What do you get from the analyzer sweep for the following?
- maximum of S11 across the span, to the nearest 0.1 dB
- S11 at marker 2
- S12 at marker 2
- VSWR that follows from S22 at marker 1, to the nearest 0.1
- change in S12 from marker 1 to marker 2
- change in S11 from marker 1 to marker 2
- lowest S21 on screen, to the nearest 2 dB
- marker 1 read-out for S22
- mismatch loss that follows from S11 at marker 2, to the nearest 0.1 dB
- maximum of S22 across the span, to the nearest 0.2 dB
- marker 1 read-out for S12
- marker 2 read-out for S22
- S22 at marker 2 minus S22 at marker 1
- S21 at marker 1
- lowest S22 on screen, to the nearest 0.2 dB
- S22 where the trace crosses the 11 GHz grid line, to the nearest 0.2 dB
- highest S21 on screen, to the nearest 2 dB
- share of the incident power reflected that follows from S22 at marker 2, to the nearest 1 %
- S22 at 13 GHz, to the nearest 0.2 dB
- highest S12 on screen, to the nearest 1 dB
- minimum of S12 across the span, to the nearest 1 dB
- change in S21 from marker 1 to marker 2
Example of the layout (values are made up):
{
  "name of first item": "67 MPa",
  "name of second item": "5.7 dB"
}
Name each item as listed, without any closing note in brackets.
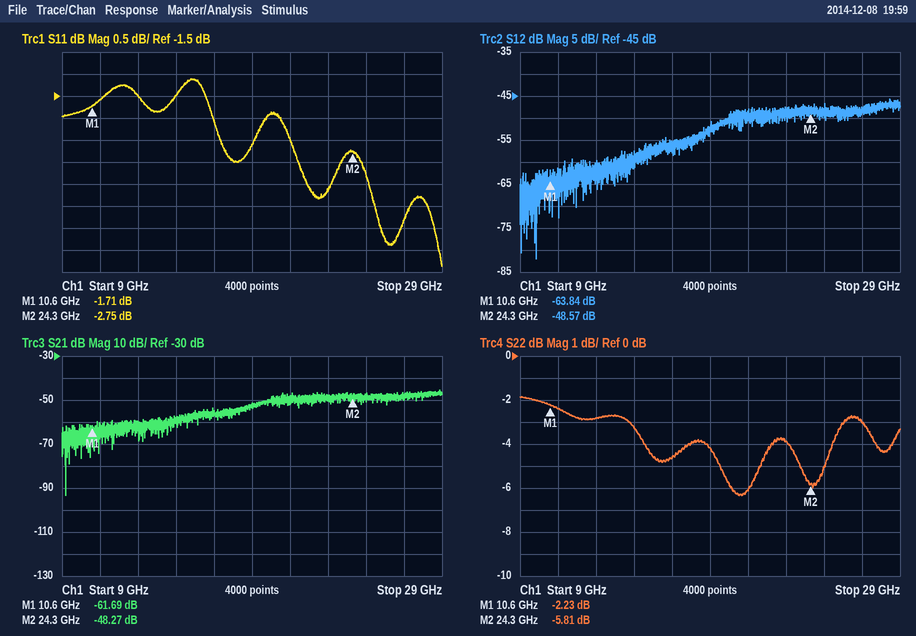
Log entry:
{
  "maximum of S11 across the span, to the nearest 0.1 dB": "-1.1 dB",
  "S11 at marker 2": "-2.75 dB",
  "S12 at marker 2": "-48.57 dB",
  "VSWR that follows from S22 at marker 1, to the nearest 0.1": "7.8",
  "change in S12 from marker 1 to marker 2": "15.27 dB",
  "change in S11 from marker 1 to marker 2": "-1.04 dB",
  "lowest S21 on screen, to the nearest 2 dB": "-94 dB",
  "marker 1 read-out for S22": "-2.23 dB",
  "mismatch loss that follows from S11 at marker 2, to the nearest 0.1 dB": "3.3 dB",
  "maximum of S22 across the span, to the nearest 0.2 dB": "-1.8 dB",
  "marker 1 read-out for S12": "-63.84 dB",
  "marker 2 read-out for S22": "-5.81 dB",
  "S22 at marker 2 minus S22 at marker 1": "-3.58 dB",
  "S21 at marker 1": "-61.69 dB",
  "lowest S22 on screen, to the nearest 0.2 dB": "-6.4 dB",
  "S22 where the trace crosses the 11 GHz grid line, to the nearest 0.2 dB": "-2.4 dB",
  "highest S21 on screen, to the nearest 2 dB": "-46 dB",
  "share of the incident power reflected that follows from S22 at marker 2, to the nearest 1 %": "26 %",
  "S22 at 13 GHz, to the nearest 0.2 dB": "-2.8 dB",
  "highest S12 on screen, to the nearest 1 dB": "-46 dB",
  "minimum of S12 across the span, to the nearest 1 dB": "-82 dB",
  "change in S21 from marker 1 to marker 2": "13.42 dB"
}
